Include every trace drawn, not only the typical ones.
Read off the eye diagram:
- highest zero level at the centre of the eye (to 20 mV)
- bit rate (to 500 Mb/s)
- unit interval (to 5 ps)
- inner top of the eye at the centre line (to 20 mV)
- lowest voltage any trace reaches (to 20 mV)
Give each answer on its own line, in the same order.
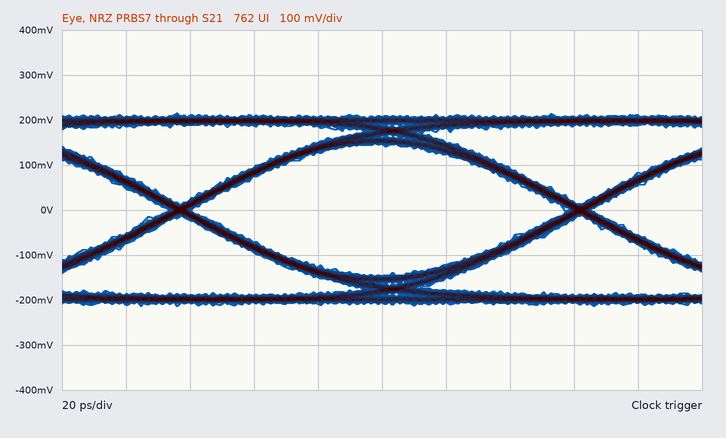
-140 mV
8.0 Gb/s
125 ps
140 mV
-220 mV
